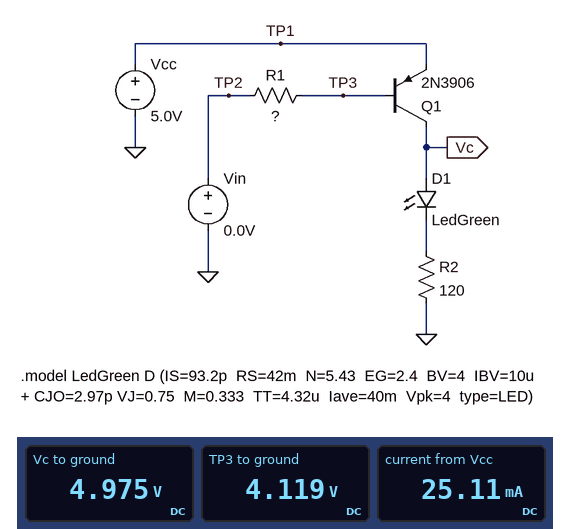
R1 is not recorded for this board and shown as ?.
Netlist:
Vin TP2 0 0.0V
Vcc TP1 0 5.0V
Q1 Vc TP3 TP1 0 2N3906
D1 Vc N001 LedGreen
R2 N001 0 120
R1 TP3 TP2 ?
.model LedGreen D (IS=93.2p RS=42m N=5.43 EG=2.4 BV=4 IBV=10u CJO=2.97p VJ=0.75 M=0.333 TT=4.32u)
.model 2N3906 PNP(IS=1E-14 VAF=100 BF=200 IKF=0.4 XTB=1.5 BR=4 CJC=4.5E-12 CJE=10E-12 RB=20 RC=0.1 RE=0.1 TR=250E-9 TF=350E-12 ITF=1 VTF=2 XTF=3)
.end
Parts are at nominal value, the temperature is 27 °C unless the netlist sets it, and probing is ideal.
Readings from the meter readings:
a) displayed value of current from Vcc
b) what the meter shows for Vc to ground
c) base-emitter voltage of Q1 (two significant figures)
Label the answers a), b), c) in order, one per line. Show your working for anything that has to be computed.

a) 25.11 mA
b) 4.975 V
c) 4.119 V - 5 V = -880 mV
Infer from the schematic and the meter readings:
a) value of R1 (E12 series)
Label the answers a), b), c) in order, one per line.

a) 680 Ω
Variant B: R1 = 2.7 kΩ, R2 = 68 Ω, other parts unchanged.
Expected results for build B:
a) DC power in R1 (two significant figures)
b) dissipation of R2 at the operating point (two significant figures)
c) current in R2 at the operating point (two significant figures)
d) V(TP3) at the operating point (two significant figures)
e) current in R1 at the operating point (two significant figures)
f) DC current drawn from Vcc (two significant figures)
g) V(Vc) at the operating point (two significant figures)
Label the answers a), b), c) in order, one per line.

a) 6.6 mW
b) 70 mW
c) 32 mA
d) 4.2 V
e) 1.6 mA
f) 34 mA
g) 4.9 V
